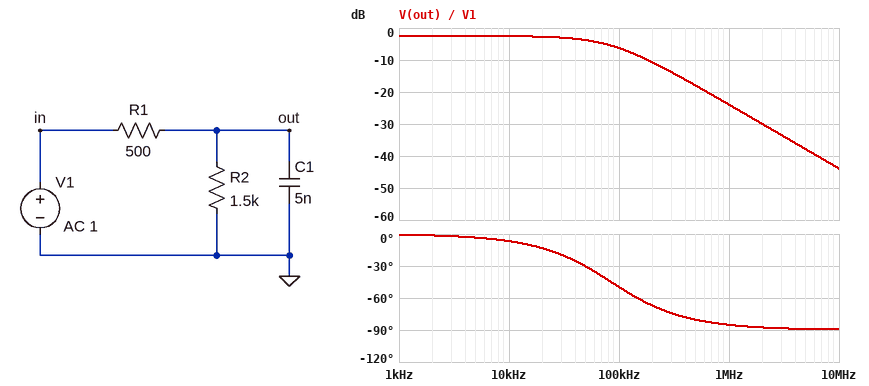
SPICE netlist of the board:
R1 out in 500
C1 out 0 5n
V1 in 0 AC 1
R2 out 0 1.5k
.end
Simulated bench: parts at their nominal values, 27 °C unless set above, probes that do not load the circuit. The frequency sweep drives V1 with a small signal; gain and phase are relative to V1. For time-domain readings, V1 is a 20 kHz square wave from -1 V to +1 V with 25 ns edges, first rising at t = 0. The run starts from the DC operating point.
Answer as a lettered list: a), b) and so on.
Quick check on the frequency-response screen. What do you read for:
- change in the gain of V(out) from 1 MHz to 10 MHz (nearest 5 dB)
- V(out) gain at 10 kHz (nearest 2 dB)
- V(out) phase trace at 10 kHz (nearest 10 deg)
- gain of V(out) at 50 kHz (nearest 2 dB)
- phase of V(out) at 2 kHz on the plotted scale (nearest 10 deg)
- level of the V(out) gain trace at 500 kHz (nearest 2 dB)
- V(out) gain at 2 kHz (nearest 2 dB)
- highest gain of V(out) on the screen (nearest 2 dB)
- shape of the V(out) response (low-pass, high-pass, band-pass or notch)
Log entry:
a) -20 dB
b) -2 dB
c) -10 deg
d) -4 dB
e) 0 deg
f) -18 dB
g) -2 dB
h) -2 dB
i) low-pass
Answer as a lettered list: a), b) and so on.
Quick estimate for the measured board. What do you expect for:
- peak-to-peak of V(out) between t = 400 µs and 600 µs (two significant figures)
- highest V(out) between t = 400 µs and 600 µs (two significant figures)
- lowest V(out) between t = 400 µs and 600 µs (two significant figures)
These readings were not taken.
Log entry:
a) 1.5 V
b) 750 mV
c) -750 mV
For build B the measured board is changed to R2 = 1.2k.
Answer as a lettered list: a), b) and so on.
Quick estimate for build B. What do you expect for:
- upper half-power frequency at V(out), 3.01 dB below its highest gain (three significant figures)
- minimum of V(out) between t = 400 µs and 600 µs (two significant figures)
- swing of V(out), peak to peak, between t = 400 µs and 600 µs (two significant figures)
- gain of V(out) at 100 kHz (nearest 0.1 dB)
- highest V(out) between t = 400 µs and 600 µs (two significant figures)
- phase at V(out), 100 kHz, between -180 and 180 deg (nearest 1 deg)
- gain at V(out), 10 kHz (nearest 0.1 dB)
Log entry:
a) 90.2 kHz
b) -710 mV
c) 1.4 V
d) -6.5 dB
e) 710 mV
f) -48 deg
g) -3.1 dB
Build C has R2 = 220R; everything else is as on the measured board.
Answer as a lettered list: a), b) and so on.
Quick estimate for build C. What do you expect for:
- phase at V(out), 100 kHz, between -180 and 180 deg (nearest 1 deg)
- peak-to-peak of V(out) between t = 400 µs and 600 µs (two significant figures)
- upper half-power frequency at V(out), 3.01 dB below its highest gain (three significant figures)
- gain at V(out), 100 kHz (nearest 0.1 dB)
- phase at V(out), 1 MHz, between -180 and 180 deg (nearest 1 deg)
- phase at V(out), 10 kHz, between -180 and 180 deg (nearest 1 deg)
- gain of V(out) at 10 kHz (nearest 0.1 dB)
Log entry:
a) -26 deg
b) 610 mV
c) 208 kHz
d) -11.2 dB
e) -78 deg
f) -3 deg
g) -10.3 dB
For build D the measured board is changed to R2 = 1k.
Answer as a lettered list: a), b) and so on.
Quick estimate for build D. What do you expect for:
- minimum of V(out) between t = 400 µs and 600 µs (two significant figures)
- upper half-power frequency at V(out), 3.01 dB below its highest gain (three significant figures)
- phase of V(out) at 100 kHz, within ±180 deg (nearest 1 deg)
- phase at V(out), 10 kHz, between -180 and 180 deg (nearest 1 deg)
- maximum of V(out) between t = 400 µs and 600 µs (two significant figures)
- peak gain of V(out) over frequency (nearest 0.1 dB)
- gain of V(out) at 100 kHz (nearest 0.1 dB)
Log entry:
a) -670 mV
b) 95.5 kHz
c) -46 deg
d) -6 deg
e) 670 mV
f) -3.5 dB
g) -6.7 dB
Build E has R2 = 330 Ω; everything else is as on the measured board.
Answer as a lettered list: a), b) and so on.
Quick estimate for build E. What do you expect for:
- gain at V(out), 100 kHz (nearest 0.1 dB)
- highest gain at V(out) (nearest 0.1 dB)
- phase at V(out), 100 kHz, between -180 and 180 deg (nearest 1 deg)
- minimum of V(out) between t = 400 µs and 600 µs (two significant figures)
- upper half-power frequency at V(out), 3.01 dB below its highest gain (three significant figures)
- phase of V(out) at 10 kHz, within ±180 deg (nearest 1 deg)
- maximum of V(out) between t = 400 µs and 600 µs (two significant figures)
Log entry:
a) -9.4 dB
b) -8.0 dB
c) -32 deg
d) -400 mV
e) 160 kHz
f) -4 deg
g) 400 mV
